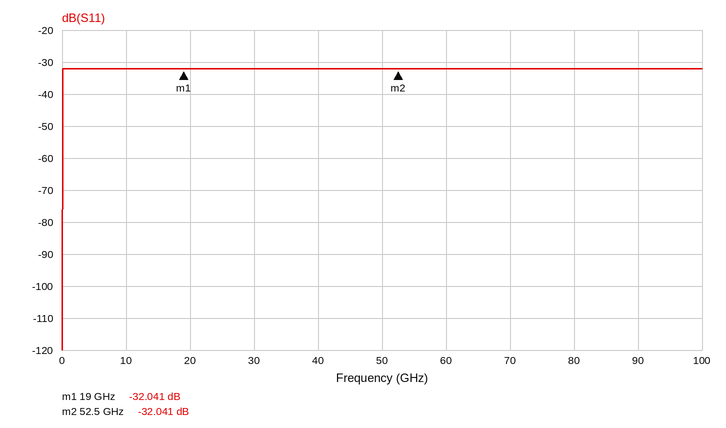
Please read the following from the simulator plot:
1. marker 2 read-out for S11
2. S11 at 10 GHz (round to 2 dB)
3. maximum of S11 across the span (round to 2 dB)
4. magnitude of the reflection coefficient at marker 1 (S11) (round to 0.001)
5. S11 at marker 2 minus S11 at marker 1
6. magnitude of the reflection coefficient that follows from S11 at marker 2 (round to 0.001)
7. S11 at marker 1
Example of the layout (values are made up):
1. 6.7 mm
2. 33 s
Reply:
1. -32.041 dB
2. -32 dB
3. -32 dB
4. 0.025
5. 0.000 dB
6. 0.025
7. -32.041 dB
